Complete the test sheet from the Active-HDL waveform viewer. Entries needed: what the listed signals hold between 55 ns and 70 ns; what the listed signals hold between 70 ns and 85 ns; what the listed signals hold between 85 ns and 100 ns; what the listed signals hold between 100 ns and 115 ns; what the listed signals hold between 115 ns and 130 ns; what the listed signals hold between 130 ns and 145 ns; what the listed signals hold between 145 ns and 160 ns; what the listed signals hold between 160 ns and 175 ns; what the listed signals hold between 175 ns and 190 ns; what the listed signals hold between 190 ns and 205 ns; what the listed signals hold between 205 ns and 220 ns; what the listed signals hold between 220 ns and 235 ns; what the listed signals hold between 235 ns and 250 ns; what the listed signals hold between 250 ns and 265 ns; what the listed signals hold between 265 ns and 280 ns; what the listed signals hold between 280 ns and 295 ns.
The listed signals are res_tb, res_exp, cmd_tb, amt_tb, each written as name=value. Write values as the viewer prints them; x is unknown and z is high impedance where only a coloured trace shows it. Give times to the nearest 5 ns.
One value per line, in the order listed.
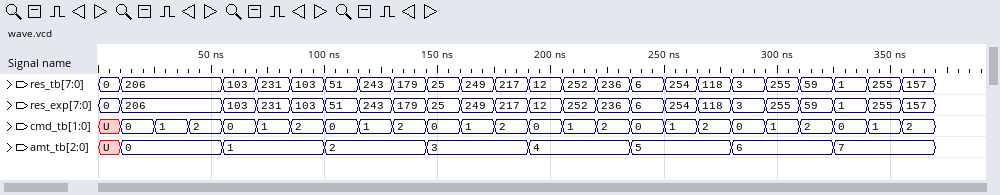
res_tb=103, res_exp=103, cmd_tb=0, amt_tb=1
res_tb=231, res_exp=231, cmd_tb=1, amt_tb=1
res_tb=103, res_exp=103, cmd_tb=2, amt_tb=1
res_tb=51, res_exp=51, cmd_tb=0, amt_tb=2
res_tb=243, res_exp=243, cmd_tb=1, amt_tb=2
res_tb=179, res_exp=179, cmd_tb=2, amt_tb=2
res_tb=25, res_exp=25, cmd_tb=0, amt_tb=3
res_tb=249, res_exp=249, cmd_tb=1, amt_tb=3
res_tb=217, res_exp=217, cmd_tb=2, amt_tb=3
res_tb=12, res_exp=12, cmd_tb=0, amt_tb=4
res_tb=252, res_exp=252, cmd_tb=1, amt_tb=4
res_tb=236, res_exp=236, cmd_tb=2, amt_tb=4
res_tb=6, res_exp=6, cmd_tb=0, amt_tb=5
res_tb=254, res_exp=254, cmd_tb=1, amt_tb=5
res_tb=118, res_exp=118, cmd_tb=2, amt_tb=5
res_tb=3, res_exp=3, cmd_tb=0, amt_tb=6
